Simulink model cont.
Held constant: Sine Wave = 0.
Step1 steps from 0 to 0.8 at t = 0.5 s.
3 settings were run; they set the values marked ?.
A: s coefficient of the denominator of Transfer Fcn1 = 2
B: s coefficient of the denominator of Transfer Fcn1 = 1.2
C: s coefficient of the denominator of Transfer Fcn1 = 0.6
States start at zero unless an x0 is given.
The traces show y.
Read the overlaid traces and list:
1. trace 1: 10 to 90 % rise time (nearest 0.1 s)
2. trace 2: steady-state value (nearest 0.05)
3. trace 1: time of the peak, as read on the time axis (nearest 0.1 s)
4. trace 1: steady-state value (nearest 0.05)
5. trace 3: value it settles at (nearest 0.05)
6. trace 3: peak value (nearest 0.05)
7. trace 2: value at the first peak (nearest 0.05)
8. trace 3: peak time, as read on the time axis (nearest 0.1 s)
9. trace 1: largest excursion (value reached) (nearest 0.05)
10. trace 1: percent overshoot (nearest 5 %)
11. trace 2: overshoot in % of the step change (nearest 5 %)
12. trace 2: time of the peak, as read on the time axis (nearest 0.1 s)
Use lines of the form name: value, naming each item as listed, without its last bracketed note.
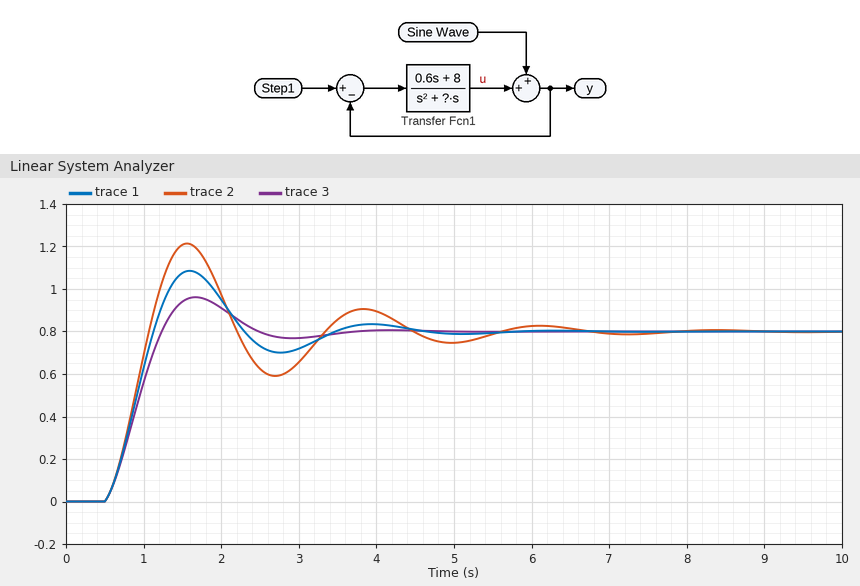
trace 1: 10 to 90 % rise time: 0.5 s
trace 2: steady-state value: 0.80
trace 1: time of the peak, as read on the time axis: 1.6 s
trace 1: steady-state value: 0.80
trace 3: value it settles at: 0.80
trace 3: peak value: 0.95
trace 2: value at the first peak: 1.20
trace 3: peak time, as read on the time axis: 1.7 s
trace 1: largest excursion (value reached): 1.10
trace 1: percent overshoot: 35 %
trace 2: overshoot in % of the step change: 50 %
trace 2: time of the peak, as read on the time axis: 1.6 s
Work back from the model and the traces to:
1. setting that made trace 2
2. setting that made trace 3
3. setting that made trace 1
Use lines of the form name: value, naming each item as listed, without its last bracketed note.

setting that made trace 2: C
setting that made trace 3: A
setting that made trace 1: B
